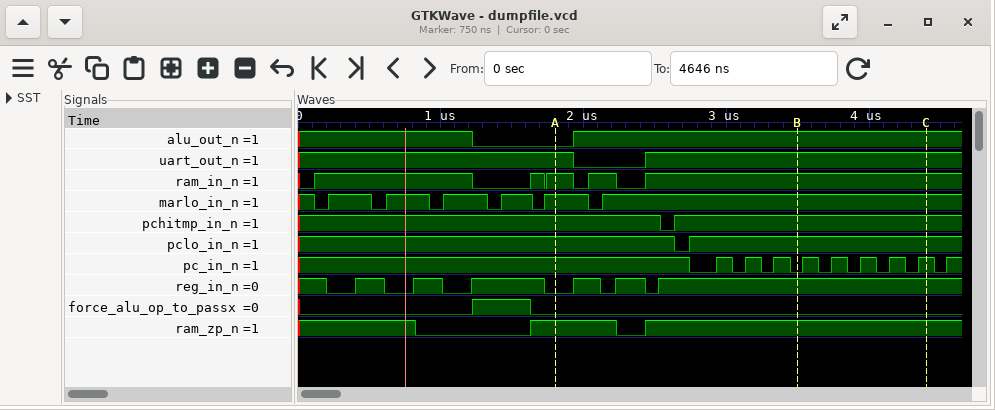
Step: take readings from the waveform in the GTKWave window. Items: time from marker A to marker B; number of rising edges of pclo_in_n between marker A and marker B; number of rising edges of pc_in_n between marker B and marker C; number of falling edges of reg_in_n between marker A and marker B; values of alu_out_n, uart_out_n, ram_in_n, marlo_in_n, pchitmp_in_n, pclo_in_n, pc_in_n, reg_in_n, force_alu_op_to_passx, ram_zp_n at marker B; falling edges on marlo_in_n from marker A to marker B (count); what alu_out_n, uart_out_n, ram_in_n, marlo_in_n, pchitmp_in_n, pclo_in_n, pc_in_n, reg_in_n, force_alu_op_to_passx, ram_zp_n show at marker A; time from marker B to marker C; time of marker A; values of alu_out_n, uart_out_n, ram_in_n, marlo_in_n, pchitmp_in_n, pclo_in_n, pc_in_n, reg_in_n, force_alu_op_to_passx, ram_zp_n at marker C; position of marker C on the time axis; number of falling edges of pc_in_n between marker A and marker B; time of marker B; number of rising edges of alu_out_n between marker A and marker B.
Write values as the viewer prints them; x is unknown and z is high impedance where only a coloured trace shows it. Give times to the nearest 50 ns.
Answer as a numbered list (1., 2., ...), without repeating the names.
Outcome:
1. 1700 ns
2. 1
3. 5
4. 2
5. alu_out_n=1, uart_out_n=1, ram_in_n=1, marlo_in_n=1, pchitmp_in_n=1, pclo_in_n=1, pc_in_n=0, reg_in_n=1, force_alu_op_to_passx=0, ram_zp_n=1
6. 1
7. alu_out_n=0, uart_out_n=1, ram_in_n=1, marlo_in_n=1, pchitmp_in_n=1, pclo_in_n=1, pc_in_n=1, reg_in_n=0, force_alu_op_to_passx=0, ram_zp_n=1
8. 900 ns
9. 1800 ns
10. alu_out_n=1, uart_out_n=1, ram_in_n=1, marlo_in_n=1, pchitmp_in_n=1, pclo_in_n=1, pc_in_n=1, reg_in_n=1, force_alu_op_to_passx=0, ram_zp_n=1
11. 4400 ns
12. 4
13. 3500 ns
14. 1
